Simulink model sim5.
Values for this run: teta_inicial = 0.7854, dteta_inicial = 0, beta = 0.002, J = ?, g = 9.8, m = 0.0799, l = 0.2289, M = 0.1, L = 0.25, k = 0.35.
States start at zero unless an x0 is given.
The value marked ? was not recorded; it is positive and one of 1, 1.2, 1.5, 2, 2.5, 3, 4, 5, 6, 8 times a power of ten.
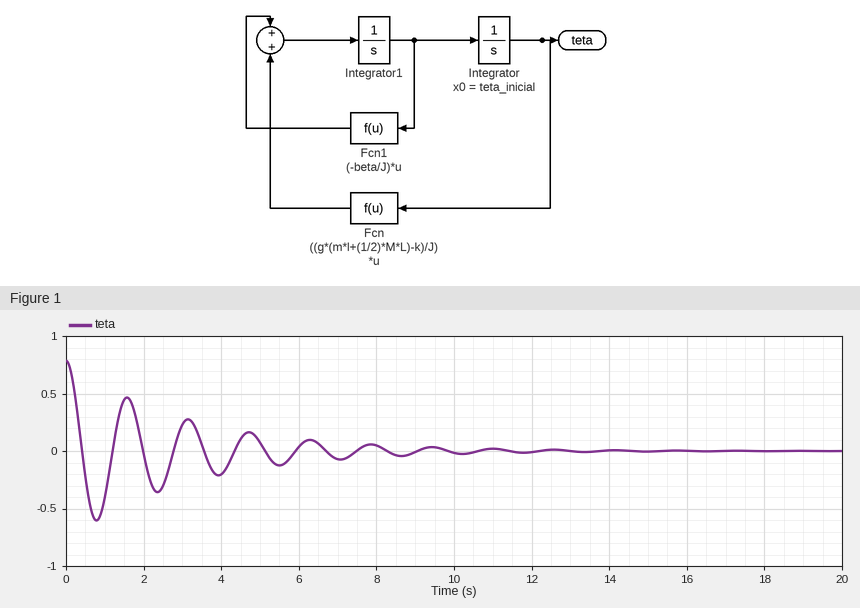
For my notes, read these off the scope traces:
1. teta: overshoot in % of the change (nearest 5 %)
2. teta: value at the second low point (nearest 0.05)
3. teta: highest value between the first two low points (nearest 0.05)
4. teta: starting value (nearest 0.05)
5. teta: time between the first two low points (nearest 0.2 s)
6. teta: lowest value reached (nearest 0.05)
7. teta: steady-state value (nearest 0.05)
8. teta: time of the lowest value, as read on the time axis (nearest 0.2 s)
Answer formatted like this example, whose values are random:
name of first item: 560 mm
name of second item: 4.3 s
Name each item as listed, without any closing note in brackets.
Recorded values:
teta: overshoot in % of the change: 75 %
teta: value at the second low point: -0.35
teta: highest value between the first two low points: 0.45
teta: starting value: 0.80
teta: time between the first two low points: 1.6 s
teta: lowest value reached: -0.60
teta: steady-state value: 0.00
teta: time of the lowest value, as read on the time axis: 0.8 s
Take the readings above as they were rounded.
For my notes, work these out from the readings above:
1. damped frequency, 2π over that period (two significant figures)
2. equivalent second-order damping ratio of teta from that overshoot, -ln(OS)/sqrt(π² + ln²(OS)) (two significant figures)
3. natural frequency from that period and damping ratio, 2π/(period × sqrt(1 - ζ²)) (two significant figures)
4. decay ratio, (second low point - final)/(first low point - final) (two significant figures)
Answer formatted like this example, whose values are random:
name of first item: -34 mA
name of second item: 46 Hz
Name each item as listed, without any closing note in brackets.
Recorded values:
damped frequency, 2π over that period: 3.9 rad/s
equivalent second-order damping ratio of teta from that overshoot, -ln(OS)/sqrt(π² + ln²(OS)): 0.091
natural frequency from that period and damping ratio, 2π/(period × sqrt(1 - ζ²)): 3.9 rad/s
decay ratio, (second low point - final)/(first low point - final): 0.58
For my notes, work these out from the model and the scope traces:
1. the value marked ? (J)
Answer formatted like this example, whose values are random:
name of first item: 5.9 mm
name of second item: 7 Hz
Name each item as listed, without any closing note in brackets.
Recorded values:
the value marked ?: 0.003
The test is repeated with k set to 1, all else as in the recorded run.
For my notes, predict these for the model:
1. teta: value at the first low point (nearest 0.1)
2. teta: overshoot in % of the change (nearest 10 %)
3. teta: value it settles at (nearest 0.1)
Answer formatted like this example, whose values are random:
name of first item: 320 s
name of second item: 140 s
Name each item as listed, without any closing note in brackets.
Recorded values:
teta: value at the first low point: -0.7
teta: overshoot in % of the change: 90 %
teta: value it settles at: 0.0
